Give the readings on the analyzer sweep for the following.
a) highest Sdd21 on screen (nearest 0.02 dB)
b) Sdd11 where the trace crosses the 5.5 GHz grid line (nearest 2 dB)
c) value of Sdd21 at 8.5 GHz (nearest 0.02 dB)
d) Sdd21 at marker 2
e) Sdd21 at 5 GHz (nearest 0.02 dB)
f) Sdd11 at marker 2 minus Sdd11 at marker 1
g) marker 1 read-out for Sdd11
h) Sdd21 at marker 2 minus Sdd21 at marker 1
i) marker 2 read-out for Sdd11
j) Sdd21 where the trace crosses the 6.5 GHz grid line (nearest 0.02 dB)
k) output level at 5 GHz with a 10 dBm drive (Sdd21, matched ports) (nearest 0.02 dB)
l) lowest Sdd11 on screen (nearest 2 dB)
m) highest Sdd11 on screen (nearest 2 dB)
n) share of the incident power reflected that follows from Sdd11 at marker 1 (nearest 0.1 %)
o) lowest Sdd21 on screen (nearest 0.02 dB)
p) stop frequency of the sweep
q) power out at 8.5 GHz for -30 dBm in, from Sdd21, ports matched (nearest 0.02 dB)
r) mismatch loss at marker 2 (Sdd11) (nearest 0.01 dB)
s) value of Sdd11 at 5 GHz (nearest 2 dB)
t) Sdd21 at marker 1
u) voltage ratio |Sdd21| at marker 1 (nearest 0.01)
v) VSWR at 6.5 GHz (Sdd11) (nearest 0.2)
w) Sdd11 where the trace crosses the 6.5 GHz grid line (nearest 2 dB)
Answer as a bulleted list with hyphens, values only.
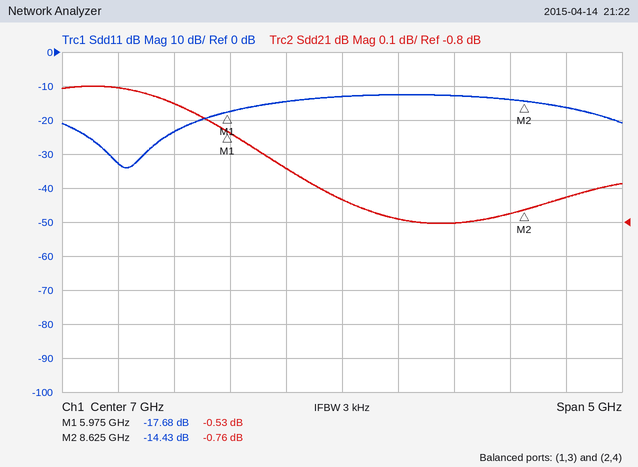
- -0.40 dB
- -24 dB
- -0.78 dB
- -0.76 dB
- -0.40 dB
- 3.25 dB
- -17.68 dB
- -0.23 dB
- -14.43 dB
- -0.64 dB
- 9.60 dBm
- -34 dB
- -12 dB
- 1.7 %
- -0.80 dB
- 9.5 GHz
- -30.78 dBm
- 0.16 dB
- -32 dB
- -0.53 dB
- 0.94
- 1.4
- -14 dB
